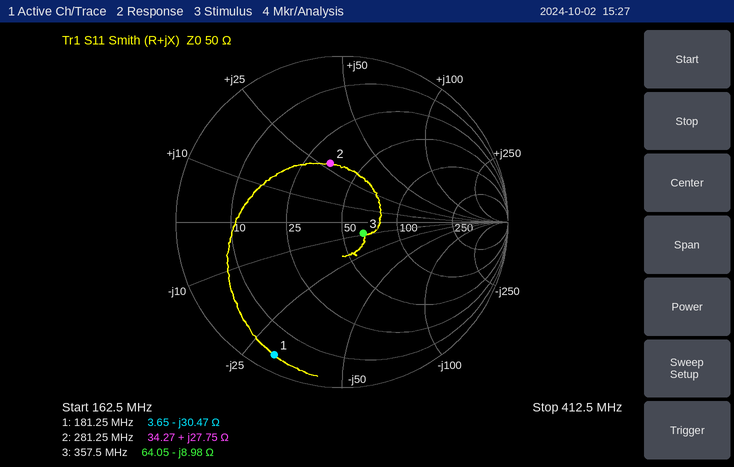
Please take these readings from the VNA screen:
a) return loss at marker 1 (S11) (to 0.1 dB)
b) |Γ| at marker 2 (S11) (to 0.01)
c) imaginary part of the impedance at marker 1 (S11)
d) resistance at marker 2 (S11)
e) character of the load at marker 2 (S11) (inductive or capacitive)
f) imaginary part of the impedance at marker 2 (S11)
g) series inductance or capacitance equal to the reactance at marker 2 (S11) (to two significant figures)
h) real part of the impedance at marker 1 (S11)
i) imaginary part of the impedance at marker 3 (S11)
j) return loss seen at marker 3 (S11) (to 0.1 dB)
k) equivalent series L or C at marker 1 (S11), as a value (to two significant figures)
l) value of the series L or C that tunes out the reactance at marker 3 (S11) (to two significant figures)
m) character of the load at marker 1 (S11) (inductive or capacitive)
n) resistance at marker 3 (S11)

0.9 dB
0.36
-30.47 Ω
34.27 Ω
inductive
+27.75 Ω
16 nH
3.65 Ω
-8.98 Ω
16.7 dB
29 pF
4.0 nH
capacitive
64.05 Ω
